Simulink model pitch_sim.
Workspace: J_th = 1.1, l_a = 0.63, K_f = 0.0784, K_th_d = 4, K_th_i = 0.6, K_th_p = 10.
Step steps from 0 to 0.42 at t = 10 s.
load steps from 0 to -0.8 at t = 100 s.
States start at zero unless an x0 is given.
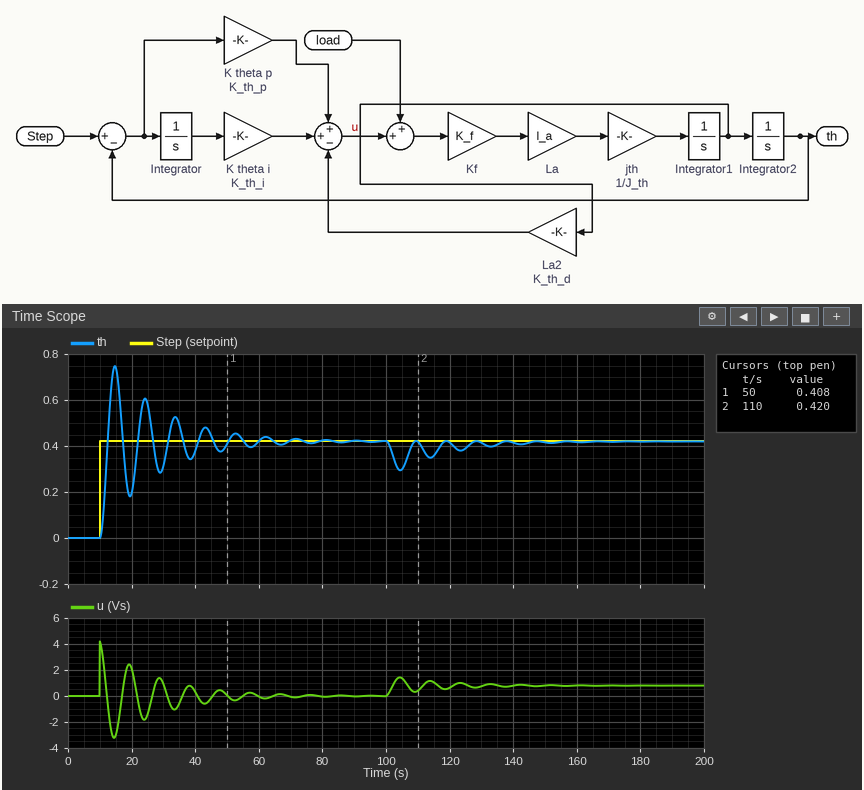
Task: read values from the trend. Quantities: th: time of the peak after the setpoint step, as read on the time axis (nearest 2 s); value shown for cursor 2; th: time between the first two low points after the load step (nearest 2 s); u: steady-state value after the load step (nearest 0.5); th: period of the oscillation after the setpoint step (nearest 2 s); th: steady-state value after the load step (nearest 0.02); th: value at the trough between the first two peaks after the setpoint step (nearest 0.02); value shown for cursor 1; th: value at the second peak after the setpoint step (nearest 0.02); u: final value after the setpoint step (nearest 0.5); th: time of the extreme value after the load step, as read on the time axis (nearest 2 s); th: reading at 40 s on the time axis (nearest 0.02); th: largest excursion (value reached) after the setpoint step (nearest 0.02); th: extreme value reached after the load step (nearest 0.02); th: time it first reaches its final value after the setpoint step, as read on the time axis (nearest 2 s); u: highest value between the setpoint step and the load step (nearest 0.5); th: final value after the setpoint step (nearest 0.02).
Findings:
14 s
0.420
10 s
1.0
10 s
0.42
0.18
0.408
0.60
0.0
104 s
0.38
0.74
0.30
12 s
4.0
0.42
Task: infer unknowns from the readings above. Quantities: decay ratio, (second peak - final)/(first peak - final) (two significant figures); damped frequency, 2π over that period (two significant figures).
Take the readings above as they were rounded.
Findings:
0.56
0.63 rad/s
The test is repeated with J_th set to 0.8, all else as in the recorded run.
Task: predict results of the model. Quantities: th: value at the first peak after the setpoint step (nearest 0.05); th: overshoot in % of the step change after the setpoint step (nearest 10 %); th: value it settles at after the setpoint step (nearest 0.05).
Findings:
0.70
70 %
0.40
